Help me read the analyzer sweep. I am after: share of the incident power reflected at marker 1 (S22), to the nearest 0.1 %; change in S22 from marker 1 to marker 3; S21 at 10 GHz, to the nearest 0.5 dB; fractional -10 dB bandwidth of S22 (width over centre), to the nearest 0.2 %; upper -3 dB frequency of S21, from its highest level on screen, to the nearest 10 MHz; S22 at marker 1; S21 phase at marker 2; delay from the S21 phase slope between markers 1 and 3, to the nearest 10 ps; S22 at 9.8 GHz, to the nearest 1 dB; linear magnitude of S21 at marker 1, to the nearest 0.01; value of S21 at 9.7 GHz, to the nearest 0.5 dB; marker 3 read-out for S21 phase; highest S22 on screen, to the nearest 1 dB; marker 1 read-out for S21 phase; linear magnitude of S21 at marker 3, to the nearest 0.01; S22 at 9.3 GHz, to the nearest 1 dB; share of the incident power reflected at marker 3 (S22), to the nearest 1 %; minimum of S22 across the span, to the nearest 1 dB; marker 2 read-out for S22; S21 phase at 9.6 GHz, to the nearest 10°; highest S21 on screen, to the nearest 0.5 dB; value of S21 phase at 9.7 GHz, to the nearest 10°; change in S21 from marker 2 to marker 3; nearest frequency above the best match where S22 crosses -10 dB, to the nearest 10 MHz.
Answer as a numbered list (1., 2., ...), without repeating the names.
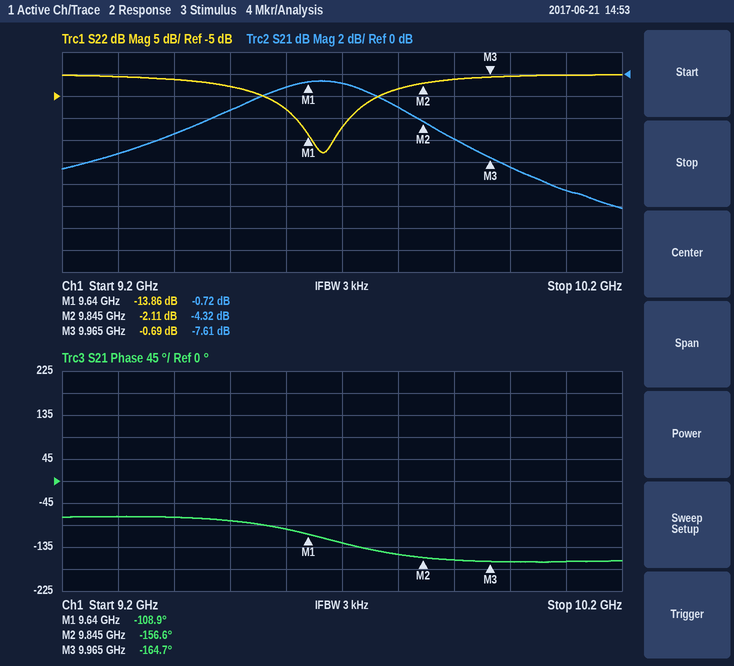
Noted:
1. 4.1 %
2. 13.17 dB
3. -8.5 dB
4. 1.0 %
5. 9.82 GHz
6. -13.86 dB
7. -156.6°
8. 480 ps
9. -3 dB
10. 0.92
11. -1.0 dB
12. -164.7°
13. 0 dB
14. -108.9°
15. 0.42
16. -1 dB
17. 85 %
18. -18 dB
19. -2.11 dB
20. -100°
21. -0.5 dB
22. -130°
23. -3.29 dB
24. 9.71 GHz
